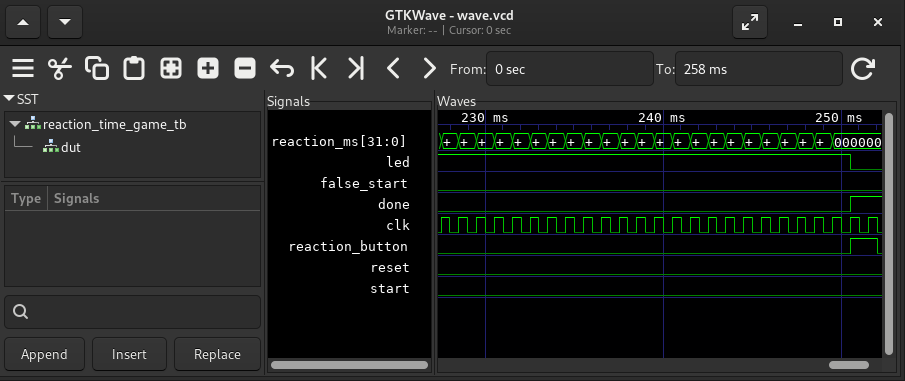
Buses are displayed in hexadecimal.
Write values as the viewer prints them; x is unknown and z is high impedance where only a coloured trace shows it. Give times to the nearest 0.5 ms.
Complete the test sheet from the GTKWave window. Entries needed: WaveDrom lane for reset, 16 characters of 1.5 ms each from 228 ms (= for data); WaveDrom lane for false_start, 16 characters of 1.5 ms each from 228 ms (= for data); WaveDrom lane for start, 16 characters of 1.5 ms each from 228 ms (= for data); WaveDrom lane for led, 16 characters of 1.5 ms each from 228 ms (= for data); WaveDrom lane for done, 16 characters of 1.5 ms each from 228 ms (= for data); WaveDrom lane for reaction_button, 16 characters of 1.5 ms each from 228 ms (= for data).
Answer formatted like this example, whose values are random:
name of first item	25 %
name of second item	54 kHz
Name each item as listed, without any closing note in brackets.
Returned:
WaveDrom lane for reset, 16 characters of 1.5 ms each from 228 ms	{name: 'reset', wave: '0...............'}
WaveDrom lane for false_start, 16 characters of 1.5 ms each from 228 ms	{name: 'false_start', wave: '0...............'}
WaveDrom lane for start, 16 characters of 1.5 ms each from 228 ms	{name: 'start', wave: '0...............'}
WaveDrom lane for led, 16 characters of 1.5 ms each from 228 ms	{name: 'led', wave: '1..............0'}
WaveDrom lane for done, 16 characters of 1.5 ms each from 228 ms	{name: 'done', wave: '0..............1'}
WaveDrom lane for reaction_button, 16 characters of 1.5 ms each from 228 ms	{name: 'reaction_button', wave: '0..............1'}
